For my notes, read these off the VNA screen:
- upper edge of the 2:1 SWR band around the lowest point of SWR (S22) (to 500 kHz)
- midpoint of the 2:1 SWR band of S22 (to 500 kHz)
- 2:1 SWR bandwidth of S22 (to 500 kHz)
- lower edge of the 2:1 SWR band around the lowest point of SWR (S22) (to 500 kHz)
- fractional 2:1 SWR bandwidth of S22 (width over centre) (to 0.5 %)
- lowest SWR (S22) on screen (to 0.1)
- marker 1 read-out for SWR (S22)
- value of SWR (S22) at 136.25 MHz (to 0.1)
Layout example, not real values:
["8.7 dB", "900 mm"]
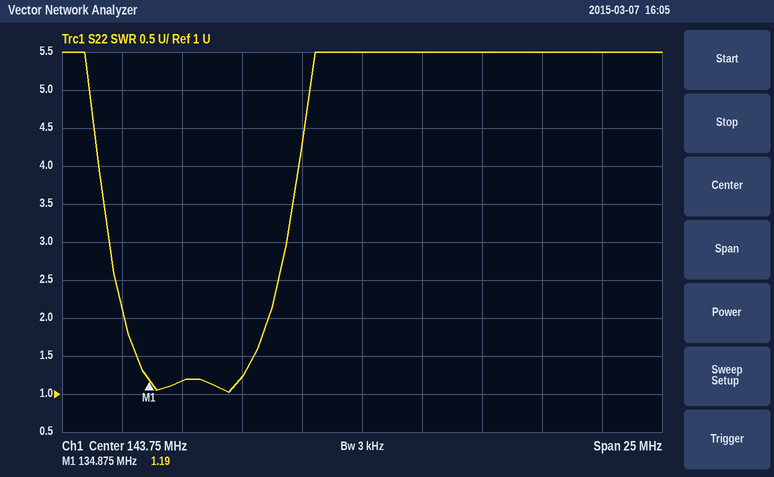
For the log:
["140.0 MHz", "137.0 MHz", "6.0 MHz", "134.0 MHz", "4.5 %", "1.0", "1.19", "1.2"]
